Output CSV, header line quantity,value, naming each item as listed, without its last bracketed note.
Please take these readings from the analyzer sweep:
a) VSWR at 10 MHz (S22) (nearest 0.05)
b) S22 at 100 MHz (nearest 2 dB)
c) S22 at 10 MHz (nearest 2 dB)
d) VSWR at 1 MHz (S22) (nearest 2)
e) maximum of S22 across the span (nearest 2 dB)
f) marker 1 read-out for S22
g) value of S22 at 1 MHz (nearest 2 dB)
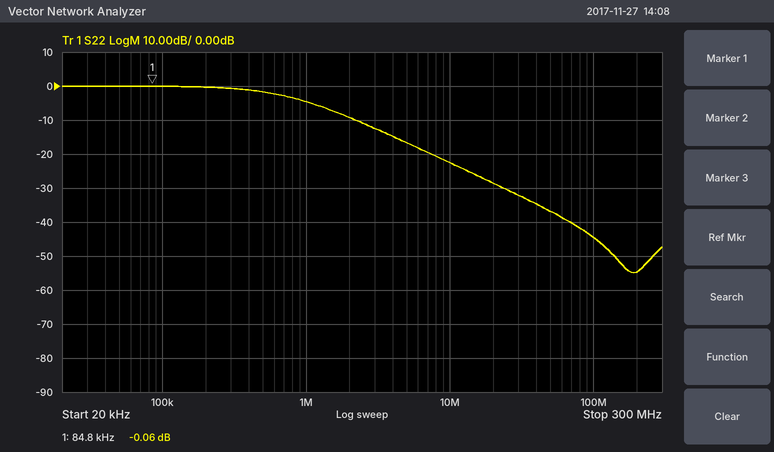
quantity,value
VSWR at 10 MHz (S22),1.15
S22 at 100 MHz,-44 dB
S22 at 10 MHz,-22 dB
VSWR at 1 MHz (S22),4
maximum of S22 across the span,0 dB
marker 1 read-out for S22,-0.06 dB
value of S22 at 1 MHz,-4 dB
